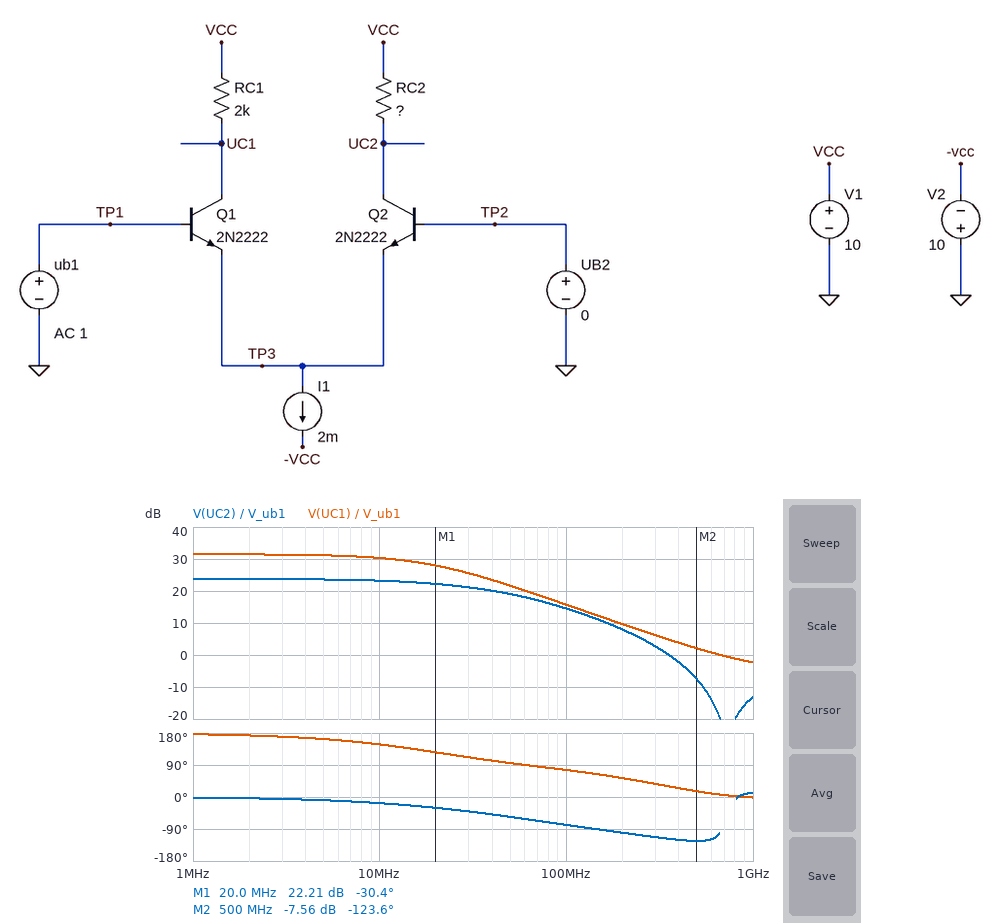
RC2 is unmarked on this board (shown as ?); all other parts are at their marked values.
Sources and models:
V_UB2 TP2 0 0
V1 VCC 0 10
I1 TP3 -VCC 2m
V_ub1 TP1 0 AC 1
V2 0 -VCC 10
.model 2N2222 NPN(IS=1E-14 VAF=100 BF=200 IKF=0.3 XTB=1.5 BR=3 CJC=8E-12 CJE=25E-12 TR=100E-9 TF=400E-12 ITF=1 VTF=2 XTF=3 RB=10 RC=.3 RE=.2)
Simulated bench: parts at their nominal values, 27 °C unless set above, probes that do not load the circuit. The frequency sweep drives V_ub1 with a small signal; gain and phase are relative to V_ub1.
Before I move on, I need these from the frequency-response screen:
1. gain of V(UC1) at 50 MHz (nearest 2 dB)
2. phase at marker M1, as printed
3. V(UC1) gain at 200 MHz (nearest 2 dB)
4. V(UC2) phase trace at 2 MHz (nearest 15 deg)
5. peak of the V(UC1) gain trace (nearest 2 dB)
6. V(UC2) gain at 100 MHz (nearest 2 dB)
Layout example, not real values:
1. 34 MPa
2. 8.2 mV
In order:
1. 22 dB
2. -30.4 deg
3. 10 dB
4. 0 deg
5. 32 dB
6. 14 dB
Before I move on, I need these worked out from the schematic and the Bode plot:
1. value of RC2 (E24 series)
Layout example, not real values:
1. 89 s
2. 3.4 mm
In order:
1. 820 Ω
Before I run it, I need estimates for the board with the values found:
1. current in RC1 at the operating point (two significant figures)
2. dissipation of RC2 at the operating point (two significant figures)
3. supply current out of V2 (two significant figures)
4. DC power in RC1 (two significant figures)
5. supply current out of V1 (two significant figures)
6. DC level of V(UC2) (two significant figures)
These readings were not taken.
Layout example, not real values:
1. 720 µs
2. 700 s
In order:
1. 990 µA
2. 820 µW
3. 2.0 mA
4. 2.0 mW
5. 2.0 mA
6. 9.2 V
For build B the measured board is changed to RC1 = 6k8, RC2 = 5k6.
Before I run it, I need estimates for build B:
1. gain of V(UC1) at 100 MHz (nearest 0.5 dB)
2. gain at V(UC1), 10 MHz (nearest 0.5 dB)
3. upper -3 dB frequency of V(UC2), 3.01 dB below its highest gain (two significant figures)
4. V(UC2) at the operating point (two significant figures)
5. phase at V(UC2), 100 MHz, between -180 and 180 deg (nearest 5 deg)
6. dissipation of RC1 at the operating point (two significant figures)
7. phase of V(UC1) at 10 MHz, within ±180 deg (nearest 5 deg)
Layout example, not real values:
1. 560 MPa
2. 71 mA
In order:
1. 13.5 dB
2. 33.0 dB
3. 4.9 MHz
4. 4.4 V
5. -100 deg
6. 6.7 mW
7. 110 deg
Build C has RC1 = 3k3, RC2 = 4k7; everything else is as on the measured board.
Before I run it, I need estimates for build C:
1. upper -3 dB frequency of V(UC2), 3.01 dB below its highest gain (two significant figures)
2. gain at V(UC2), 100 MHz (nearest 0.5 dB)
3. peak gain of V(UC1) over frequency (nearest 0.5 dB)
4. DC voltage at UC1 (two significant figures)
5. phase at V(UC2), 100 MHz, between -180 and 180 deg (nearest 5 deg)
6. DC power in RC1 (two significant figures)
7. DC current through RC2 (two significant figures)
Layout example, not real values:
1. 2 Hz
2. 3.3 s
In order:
1. 6.6 MHz
2. 14.0 dB
3. 35.5 dB
4. 6.7 V
5. -100 deg
6. 3.3 mW
7. 990 µA
